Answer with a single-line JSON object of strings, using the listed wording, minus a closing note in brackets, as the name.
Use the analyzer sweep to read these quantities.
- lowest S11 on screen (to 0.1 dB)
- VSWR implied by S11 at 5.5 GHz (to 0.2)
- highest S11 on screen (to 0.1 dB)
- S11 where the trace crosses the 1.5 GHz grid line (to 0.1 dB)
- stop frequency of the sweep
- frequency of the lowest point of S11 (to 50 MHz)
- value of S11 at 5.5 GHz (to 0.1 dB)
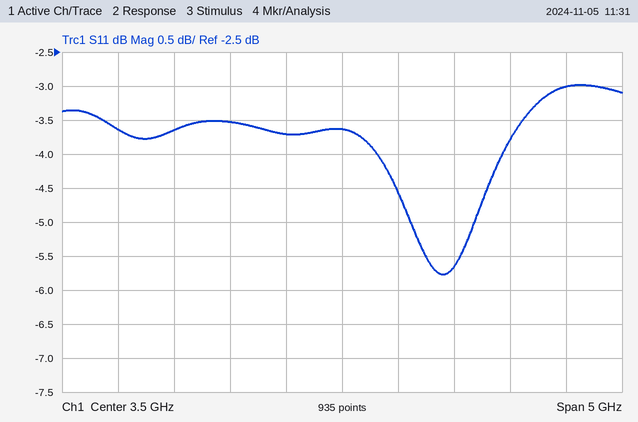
{"lowest S11 on screen": "-5.8 dB", "VSWR implied by S11 at 5.5 GHz": "5.8", "highest S11 on screen": "-3.0 dB", "S11 where the trace crosses the 1.5 GHz grid line": "-3.6 dB", "stop frequency of the sweep": "6 GHz", "frequency of the lowest point of S11": "4.40 GHz", "value of S11 at 5.5 GHz": "-3.0 dB"}
